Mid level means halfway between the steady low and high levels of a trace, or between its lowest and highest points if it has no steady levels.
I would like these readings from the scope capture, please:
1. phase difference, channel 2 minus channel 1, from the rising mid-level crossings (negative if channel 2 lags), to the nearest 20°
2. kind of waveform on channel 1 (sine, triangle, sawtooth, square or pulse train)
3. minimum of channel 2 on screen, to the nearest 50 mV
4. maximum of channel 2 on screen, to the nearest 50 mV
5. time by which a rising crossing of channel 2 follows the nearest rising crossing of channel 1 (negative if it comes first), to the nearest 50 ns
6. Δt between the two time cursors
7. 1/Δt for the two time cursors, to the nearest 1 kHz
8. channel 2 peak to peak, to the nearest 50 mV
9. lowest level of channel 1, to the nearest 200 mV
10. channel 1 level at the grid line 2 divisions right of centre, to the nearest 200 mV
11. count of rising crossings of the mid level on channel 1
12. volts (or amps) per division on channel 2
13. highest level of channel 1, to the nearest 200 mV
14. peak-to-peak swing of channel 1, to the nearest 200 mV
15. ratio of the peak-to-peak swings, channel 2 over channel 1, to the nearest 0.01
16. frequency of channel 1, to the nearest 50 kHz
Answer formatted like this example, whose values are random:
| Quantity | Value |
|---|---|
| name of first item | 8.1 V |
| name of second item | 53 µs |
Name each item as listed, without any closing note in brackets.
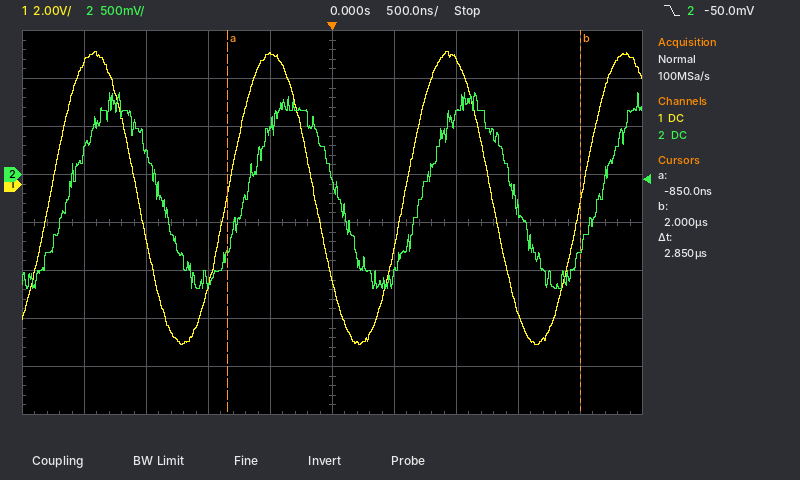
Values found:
| Quantity | Value |
|---|---|
| phase difference, channel 2 minus channel 1, from the rising mid-level crossings (negative if channel 2 lags), to the nearest 20° | -40° |
| kind of waveform on channel 1 | sine |
| minimum of channel 2 on screen, to the nearest 50 mV | -1.20 V |
| maximum of channel 2 on screen, to the nearest 50 mV | 850 mV |
| time by which a rising crossing of channel 2 follows the nearest rising crossing of channel 1 (negative if it comes first), to the nearest 50 ns | +150 ns |
| Δt between the two time cursors | 2.85 µs |
| 1/Δt for the two time cursors, to the nearest 1 kHz | 351 kHz |
| channel 2 peak to peak, to the nearest 50 mV | 2.05 V |
| lowest level of channel 1, to the nearest 200 mV | -6.6 V |
| channel 1 level at the grid line 2 divisions right of centre, to the nearest 200 mV | 5.2 V |
| count of rising crossings of the mid level on channel 1 | 4 |
| volts (or amps) per division on channel 2 | 500 mV |
| highest level of channel 1, to the nearest 200 mV | 5.6 V |
| peak-to-peak swing of channel 1, to the nearest 200 mV | 12.2 V |
| ratio of the peak-to-peak swings, channel 2 over channel 1, to the nearest 0.01 | 0.17 |
| frequency of channel 1, to the nearest 50 kHz | 700 kHz |
